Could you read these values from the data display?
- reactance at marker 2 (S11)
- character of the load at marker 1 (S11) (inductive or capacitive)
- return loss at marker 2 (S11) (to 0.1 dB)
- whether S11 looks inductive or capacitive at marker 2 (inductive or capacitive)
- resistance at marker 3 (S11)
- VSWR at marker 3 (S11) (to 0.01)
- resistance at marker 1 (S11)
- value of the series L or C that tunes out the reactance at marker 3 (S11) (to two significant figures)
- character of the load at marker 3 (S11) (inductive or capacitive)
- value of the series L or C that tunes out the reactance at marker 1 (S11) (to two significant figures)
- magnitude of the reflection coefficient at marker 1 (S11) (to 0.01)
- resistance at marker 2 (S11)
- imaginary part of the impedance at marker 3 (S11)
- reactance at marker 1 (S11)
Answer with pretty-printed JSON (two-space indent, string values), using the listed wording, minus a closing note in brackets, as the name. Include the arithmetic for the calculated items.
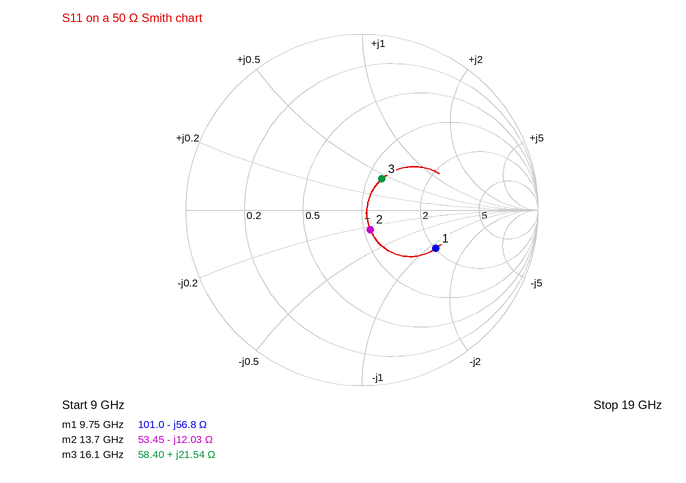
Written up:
{
  "reactance at marker 2": "-12.03 Ω",
  "character of the load at marker 1 (S11)": "capacitive",
  "return loss at marker 2 (S11)": "18.4 dB",
  "whether S11 looks inductive or capacitive at marker 2": "capacitive",
  "resistance at marker 3": "58.40 Ω",
  "VSWR at marker 3 (S11)": "1.53",
  "resistance at marker 1": "101.0 Ω",
  "value of the series L or C that tunes out the reactance at marker 3 (S11)": "C = 1/(2π × 16.1 GHz × 21.54 Ω) ≈ 459 fF, so 460 fF to two significant figures",
  "character of the load at marker 3 (S11)": "inductive",
  "value of the series L or C that tunes out the reactance at marker 1 (S11)": "L = 56.8 Ω/(2π × 9.75 GHz) ≈ 927 pH, so 930 pH to two significant figures",
  "magnitude of the reflection coefficient at marker 1 (S11)": "0.47",
  "resistance at marker 2": "53.45 Ω",
  "imaginary part of the impedance at marker 3": "+21.54 Ω",
  "reactance at marker 1": "-56.8 Ω"
}
